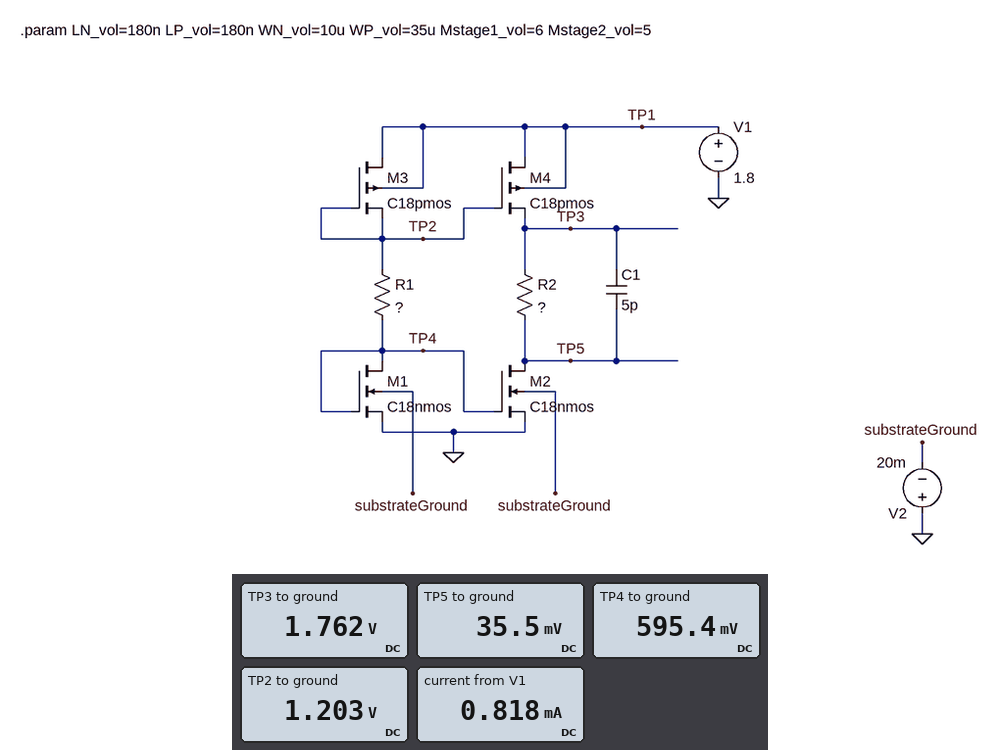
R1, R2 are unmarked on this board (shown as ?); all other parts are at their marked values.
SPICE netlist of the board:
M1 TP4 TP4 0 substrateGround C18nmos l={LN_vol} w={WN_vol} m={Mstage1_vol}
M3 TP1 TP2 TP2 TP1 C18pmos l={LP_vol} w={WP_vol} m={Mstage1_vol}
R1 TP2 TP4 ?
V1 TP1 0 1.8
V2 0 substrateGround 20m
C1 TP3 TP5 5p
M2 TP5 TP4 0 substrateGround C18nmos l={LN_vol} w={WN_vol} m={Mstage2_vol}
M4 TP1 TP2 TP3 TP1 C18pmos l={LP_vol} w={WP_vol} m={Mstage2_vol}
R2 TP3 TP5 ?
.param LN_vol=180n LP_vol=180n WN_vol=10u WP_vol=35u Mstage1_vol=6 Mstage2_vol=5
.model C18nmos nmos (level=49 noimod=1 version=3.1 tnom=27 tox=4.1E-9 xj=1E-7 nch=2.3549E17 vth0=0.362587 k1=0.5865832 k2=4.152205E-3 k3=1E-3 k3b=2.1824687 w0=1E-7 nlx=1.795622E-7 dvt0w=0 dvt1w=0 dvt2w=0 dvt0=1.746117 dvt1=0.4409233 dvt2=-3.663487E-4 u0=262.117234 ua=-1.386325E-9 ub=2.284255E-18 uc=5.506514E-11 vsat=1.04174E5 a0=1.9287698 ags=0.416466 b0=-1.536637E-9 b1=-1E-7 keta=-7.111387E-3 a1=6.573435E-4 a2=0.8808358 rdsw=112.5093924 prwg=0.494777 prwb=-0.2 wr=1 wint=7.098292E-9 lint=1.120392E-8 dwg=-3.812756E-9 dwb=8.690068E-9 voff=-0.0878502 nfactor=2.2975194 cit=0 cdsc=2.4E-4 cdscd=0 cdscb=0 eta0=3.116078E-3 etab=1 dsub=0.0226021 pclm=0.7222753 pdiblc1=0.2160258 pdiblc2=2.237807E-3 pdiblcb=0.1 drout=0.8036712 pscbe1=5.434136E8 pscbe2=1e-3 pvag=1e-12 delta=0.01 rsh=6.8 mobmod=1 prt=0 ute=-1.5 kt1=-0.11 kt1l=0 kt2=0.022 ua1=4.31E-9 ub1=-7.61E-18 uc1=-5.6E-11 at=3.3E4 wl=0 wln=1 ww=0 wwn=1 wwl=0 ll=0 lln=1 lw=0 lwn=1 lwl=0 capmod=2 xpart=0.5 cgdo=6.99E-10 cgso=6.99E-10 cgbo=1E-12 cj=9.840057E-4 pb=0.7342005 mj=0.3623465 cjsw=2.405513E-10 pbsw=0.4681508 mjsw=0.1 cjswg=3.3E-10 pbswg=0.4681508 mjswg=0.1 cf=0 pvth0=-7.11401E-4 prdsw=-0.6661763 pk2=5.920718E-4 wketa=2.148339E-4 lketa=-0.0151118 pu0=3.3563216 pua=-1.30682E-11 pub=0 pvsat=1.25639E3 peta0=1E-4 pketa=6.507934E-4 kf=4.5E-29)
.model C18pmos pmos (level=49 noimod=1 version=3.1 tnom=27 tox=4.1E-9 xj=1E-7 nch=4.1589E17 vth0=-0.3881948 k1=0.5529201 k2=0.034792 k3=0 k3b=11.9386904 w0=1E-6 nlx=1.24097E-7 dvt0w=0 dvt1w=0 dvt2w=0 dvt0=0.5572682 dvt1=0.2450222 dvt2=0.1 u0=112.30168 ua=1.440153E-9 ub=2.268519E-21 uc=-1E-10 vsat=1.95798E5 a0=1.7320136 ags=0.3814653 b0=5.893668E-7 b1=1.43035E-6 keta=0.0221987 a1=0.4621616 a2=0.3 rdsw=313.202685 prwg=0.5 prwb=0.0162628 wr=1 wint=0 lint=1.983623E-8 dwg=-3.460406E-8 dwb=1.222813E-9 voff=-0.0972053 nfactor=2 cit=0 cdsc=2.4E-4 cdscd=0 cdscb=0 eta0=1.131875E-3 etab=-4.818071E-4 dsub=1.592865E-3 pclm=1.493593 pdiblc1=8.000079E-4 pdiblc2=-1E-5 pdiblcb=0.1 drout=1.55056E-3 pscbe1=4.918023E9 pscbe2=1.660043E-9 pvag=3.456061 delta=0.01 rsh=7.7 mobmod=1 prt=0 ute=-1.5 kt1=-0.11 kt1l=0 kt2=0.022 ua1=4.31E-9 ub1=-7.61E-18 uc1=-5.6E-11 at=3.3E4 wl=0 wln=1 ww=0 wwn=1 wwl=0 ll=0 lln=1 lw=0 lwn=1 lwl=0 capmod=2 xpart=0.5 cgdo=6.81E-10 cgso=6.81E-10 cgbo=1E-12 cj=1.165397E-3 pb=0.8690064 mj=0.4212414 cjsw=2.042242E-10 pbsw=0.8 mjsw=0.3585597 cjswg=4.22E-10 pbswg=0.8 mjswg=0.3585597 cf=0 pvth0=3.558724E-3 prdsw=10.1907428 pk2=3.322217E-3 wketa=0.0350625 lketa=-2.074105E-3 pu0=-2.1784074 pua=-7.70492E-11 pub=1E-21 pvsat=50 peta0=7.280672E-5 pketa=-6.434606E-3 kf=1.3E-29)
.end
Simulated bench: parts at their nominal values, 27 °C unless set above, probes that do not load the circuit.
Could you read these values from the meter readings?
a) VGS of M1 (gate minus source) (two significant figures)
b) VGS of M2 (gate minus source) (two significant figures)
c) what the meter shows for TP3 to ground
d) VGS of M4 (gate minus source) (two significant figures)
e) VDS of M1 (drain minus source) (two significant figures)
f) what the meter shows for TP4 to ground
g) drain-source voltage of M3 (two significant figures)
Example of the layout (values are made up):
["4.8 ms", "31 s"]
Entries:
["600 mV", "600 mV", "1.762 V", "-560 mV", "600 mV", "595.4 mV", "600 mV"]
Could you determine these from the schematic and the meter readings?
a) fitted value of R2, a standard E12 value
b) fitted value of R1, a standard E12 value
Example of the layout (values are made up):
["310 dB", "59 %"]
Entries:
["8.2 kΩ", "1 kΩ"]
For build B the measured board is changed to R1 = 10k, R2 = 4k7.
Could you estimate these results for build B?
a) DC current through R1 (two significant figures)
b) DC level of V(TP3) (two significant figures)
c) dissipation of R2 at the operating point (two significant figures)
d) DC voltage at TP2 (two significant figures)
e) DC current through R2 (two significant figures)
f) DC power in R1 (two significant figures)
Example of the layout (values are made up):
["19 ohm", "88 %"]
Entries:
["82 µA", "1.0 V", "25 µW", "1.3 V", "73 µA", "67 µW"]
